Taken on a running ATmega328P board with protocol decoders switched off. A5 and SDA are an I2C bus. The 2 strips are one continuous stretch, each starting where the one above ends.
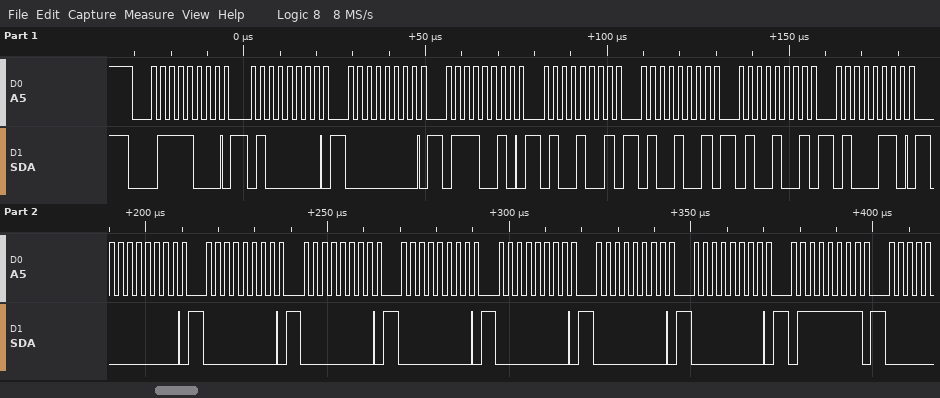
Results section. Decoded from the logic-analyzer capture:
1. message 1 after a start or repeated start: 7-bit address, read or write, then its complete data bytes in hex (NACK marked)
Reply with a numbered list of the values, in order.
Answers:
1. 0x3C write: 40 00 72 49 49 49 46 00 00 00 00 00 00 00 7F
